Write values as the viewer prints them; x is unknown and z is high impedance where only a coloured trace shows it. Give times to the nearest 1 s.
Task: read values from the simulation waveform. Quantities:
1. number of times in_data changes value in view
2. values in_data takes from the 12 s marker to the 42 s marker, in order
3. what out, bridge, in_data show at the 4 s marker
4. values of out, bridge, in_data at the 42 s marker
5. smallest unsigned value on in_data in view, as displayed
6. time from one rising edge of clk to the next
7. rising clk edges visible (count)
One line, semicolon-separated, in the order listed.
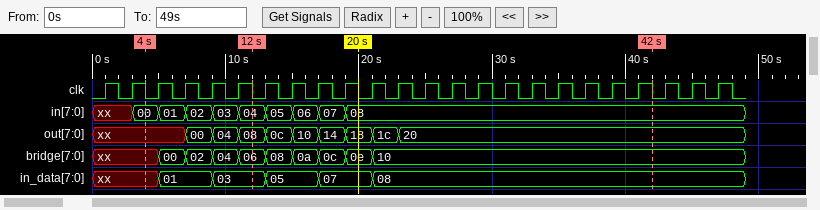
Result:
5; 03, 05, 07, 08; out=xx, bridge=xx, in_data=xx; out=20, bridge=10, in_data=08; 01; 2 s; 24
